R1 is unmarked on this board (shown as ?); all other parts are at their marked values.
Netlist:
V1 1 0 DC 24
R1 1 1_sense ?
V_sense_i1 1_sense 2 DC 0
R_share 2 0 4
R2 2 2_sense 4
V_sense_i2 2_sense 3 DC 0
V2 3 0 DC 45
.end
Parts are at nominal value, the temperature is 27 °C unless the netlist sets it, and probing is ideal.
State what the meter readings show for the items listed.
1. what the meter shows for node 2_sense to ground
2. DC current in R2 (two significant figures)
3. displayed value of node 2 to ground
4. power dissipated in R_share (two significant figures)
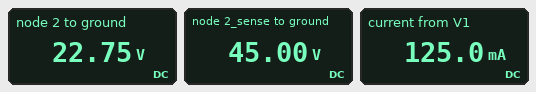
45.00 V
5.6 A
22.75 V
130 W
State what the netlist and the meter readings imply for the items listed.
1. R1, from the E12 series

10 Ω
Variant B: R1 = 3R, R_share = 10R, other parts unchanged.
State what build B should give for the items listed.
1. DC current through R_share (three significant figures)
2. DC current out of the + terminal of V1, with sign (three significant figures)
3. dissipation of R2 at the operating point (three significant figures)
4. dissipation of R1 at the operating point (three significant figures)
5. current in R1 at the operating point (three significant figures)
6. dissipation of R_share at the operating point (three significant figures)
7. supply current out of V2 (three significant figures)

2.82 A
-1.39 A
70.8 W
5.80 W
1.39 A
79.4 W
4.21 A
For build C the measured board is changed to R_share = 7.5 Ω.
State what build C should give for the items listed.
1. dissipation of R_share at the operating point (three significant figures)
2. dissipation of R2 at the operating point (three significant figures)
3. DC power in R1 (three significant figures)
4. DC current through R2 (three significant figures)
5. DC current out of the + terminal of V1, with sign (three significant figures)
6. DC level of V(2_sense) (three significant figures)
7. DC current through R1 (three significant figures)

106 W
70.2 W
1.80 W
4.19 A
-424 mA
45.0 V
424 mA
